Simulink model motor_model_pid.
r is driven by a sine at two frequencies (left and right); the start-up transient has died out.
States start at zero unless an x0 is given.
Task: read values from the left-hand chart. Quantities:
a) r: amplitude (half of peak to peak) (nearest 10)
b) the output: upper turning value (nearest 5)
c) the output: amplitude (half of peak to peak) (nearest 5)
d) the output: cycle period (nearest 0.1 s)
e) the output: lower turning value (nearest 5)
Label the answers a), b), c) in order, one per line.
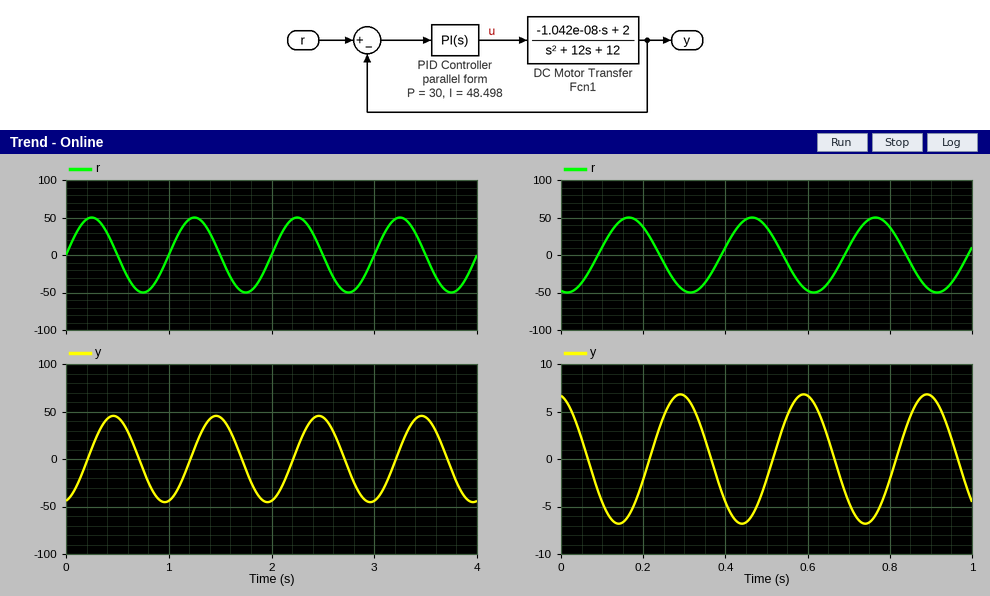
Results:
a) 50
b) 45
c) 45
d) 1.0 s
e) -45
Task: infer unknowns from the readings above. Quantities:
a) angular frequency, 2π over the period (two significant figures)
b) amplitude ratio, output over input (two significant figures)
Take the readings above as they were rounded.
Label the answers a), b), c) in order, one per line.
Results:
a) 6.3 rad/s
b) 0.90
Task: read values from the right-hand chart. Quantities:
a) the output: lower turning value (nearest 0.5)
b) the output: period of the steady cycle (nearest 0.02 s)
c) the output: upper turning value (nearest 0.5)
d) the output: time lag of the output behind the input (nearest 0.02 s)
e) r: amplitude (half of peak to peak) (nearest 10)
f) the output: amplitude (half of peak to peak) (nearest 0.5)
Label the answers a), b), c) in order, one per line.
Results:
a) -7.0
b) 0.30 s
c) 7.0
d) 0.12 s
e) 50
f) 7.0
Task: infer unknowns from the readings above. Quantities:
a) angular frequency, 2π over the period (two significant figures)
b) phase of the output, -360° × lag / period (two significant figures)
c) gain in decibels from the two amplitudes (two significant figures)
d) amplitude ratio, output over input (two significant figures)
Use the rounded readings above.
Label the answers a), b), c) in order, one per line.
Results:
a) 21 rad/s
b) -140°
c) -17 dB
d) 0.14
